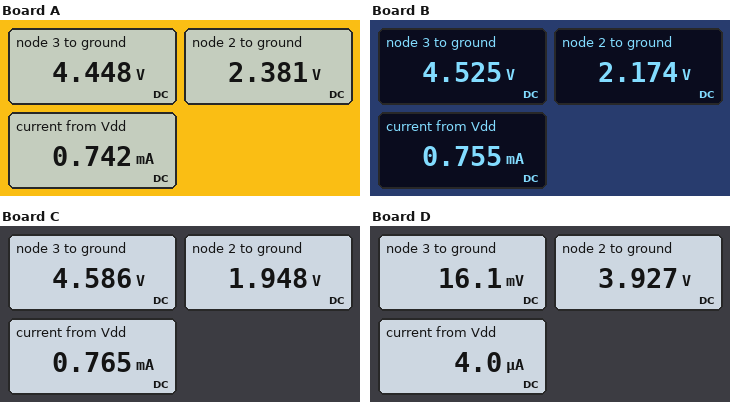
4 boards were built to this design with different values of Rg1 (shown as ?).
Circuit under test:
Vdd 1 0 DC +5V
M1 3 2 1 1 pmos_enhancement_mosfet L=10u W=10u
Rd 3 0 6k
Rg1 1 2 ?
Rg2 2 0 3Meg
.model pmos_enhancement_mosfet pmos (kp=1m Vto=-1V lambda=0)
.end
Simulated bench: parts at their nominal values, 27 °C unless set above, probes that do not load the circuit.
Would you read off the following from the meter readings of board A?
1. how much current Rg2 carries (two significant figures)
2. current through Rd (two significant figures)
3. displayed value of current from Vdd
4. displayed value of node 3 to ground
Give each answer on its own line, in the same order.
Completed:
790 nA
740 µA
0.742 mA
4.448 V
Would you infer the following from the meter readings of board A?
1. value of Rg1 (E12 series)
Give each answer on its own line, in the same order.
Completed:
3.3 MΩ
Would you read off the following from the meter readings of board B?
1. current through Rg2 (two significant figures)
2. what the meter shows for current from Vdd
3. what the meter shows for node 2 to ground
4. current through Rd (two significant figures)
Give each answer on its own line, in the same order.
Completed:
720 nA
0.755 mA
2.174 V
750 µA
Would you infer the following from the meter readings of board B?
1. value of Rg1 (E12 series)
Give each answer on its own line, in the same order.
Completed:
3.9 MΩ
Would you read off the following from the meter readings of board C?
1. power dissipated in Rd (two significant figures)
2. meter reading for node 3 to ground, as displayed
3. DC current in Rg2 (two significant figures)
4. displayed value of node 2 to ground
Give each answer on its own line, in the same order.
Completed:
3.5 mW
4.586 V
650 nA
1.948 V
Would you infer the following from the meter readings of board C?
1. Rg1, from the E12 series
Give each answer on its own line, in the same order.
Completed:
4.7 MΩ
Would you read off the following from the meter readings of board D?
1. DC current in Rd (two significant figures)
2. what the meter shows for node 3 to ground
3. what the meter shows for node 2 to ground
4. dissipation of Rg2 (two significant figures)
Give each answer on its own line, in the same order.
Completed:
2.7 µA
16.1 mV
3.927 V
5.1 µW
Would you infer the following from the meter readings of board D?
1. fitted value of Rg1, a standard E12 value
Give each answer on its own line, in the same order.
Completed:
820 kΩ
